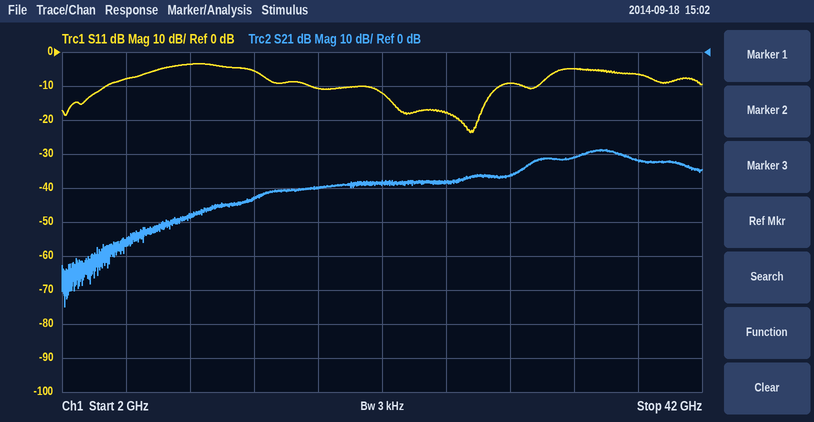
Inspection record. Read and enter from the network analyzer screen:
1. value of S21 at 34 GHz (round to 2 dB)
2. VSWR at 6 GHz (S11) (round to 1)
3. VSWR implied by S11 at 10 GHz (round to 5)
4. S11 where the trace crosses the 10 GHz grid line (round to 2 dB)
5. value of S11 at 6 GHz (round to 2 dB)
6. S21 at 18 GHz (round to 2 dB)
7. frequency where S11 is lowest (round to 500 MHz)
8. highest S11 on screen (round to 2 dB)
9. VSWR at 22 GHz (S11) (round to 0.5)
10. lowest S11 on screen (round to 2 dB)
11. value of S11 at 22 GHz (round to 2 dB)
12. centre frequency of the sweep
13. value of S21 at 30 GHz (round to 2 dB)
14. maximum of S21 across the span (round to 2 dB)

-30 dB
2
5
-4 dB
-8 dB
-40 dB
27.5 GHz
-4 dB
1.5
-24 dB
-12 dB
22 GHz
-36 dB
-28 dB
